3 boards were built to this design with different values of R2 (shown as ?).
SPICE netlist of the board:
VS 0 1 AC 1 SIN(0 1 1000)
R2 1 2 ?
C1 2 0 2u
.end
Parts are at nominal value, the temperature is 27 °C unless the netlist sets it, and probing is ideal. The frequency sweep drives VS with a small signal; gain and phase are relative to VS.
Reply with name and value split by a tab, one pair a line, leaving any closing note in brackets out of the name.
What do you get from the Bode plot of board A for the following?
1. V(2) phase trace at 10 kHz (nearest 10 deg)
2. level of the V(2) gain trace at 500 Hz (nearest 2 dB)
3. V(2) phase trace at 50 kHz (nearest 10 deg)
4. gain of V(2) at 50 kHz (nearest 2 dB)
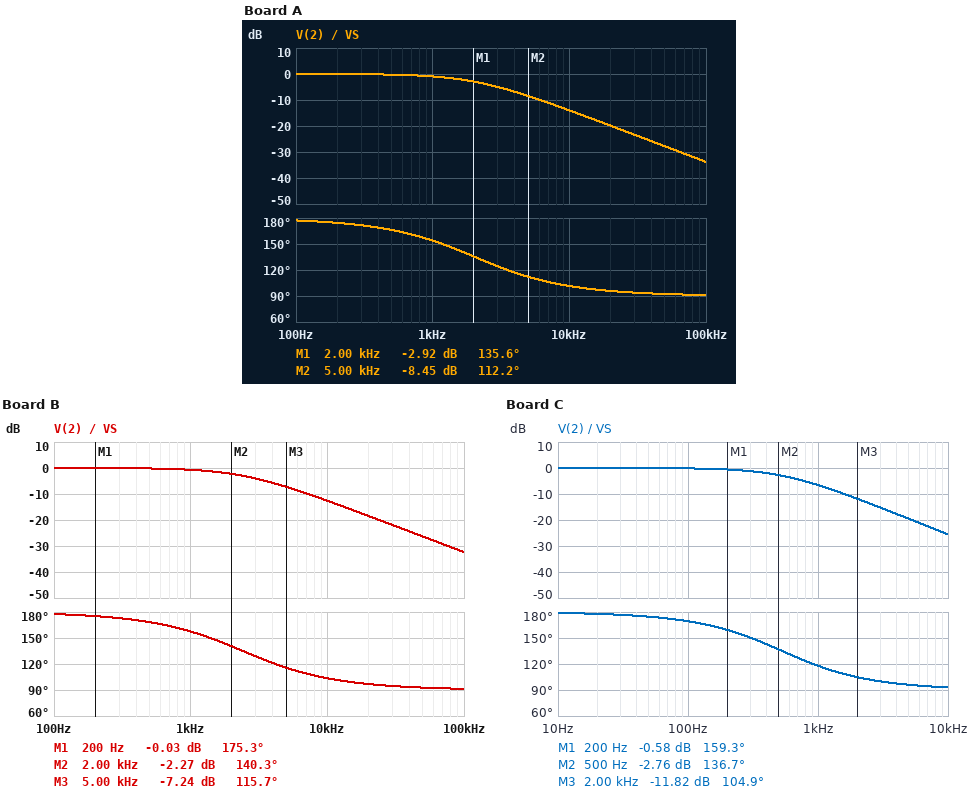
V(2) phase trace at 10 kHz	100 deg
level of the V(2) gain trace at 500 Hz	0 dB
V(2) phase trace at 50 kHz	90 deg
gain of V(2) at 50 kHz	-28 dB
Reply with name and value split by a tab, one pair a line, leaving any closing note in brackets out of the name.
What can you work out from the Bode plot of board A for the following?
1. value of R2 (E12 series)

value of R2	39 Ω
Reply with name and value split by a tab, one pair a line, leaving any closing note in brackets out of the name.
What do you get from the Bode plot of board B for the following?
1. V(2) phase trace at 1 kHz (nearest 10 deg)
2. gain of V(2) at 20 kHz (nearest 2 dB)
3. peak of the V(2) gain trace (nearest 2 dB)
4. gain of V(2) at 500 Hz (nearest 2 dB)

V(2) phase trace at 1 kHz	160 deg
gain of V(2) at 20 kHz	-18 dB
peak of the V(2) gain trace	0 dB
gain of V(2) at 500 Hz	0 dB
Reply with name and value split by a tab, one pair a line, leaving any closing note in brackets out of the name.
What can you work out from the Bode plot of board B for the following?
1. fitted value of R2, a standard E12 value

fitted value of R2, a standard E12 value	33 Ω
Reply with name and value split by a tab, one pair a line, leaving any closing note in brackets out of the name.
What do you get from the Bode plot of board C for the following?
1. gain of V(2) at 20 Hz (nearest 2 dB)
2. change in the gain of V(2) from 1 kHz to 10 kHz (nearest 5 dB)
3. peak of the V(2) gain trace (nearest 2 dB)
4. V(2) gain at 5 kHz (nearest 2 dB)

gain of V(2) at 20 Hz	0 dB
change in the gain of V(2) from 1 kHz to 10 kHz	-20 dB
peak of the V(2) gain trace	0 dB
V(2) gain at 5 kHz	-20 dB
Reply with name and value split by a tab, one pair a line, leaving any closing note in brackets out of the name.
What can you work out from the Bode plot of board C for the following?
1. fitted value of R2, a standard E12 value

fitted value of R2, a standard E12 value	150 Ω
